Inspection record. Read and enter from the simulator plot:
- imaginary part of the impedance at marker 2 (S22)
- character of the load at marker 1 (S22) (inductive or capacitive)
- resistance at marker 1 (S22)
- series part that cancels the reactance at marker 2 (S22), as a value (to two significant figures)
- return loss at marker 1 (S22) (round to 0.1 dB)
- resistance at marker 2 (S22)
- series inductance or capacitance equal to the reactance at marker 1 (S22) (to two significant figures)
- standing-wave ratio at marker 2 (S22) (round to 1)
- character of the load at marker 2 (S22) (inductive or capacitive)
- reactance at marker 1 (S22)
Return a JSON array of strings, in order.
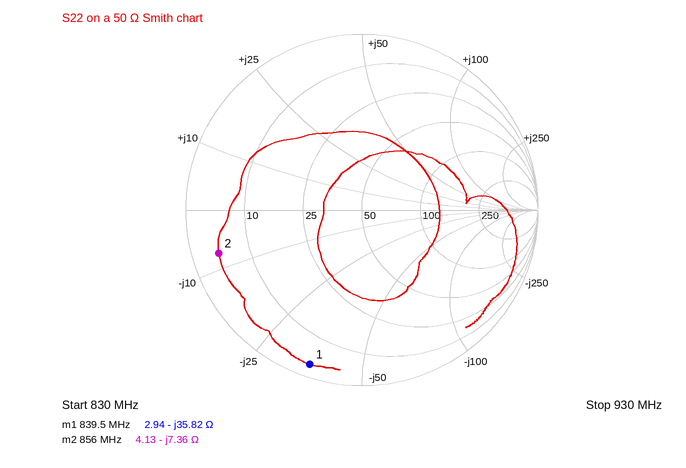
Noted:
["-7.36 Ω", "capacitive", "2.94 Ω", "1.4 nH", "0.7 dB", "4.13 Ω", "5.3 pF", "12", "capacitive", "-35.82 Ω"]
